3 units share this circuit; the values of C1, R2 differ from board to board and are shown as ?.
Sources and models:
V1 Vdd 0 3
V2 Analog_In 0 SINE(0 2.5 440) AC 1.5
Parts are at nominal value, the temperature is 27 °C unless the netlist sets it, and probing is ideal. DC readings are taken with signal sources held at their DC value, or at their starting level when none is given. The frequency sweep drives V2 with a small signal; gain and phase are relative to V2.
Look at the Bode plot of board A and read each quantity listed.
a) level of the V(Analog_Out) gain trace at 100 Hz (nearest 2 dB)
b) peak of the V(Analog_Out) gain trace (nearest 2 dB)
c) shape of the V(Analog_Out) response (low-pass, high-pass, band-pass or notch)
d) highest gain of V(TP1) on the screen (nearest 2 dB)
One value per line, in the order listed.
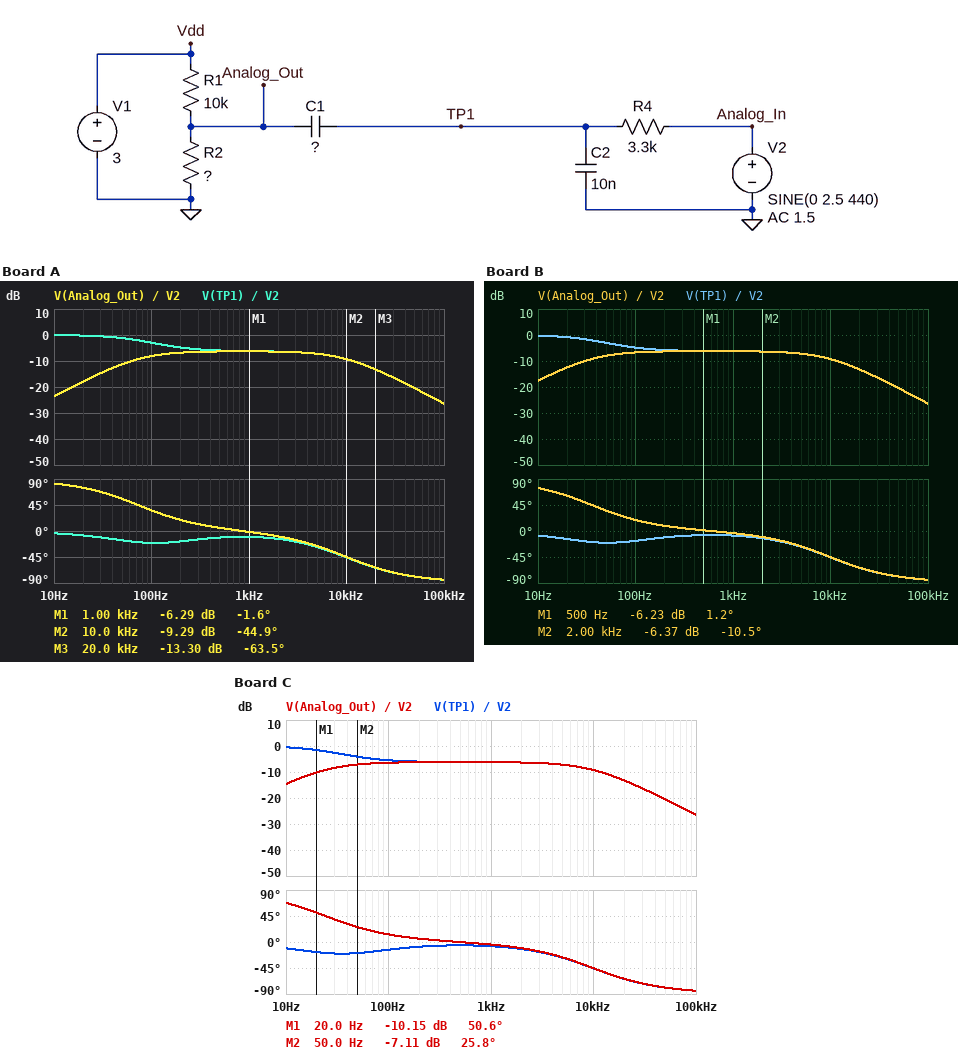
-8 dB
-6 dB
band-pass
0 dB
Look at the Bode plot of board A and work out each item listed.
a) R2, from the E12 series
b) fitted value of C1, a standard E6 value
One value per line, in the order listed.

4.7 kΩ
330 nF
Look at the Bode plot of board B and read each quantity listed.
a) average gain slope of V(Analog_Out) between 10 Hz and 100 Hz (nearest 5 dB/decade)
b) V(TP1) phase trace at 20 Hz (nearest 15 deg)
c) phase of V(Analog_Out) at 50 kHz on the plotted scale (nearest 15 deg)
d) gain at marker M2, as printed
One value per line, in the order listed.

10 dB/decade
-15 deg
-75 deg
-6.37 dB
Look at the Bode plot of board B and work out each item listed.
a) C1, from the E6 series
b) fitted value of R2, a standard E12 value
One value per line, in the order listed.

680 nF
4.7 kΩ
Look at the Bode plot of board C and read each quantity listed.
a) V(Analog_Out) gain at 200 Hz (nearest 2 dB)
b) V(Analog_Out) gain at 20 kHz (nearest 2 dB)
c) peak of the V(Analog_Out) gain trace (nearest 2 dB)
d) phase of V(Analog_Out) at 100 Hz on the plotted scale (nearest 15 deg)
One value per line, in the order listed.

-6 dB
-14 dB
-6 dB
15 deg
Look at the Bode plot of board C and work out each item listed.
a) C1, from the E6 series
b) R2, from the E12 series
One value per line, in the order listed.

1 µF
4.7 kΩ
